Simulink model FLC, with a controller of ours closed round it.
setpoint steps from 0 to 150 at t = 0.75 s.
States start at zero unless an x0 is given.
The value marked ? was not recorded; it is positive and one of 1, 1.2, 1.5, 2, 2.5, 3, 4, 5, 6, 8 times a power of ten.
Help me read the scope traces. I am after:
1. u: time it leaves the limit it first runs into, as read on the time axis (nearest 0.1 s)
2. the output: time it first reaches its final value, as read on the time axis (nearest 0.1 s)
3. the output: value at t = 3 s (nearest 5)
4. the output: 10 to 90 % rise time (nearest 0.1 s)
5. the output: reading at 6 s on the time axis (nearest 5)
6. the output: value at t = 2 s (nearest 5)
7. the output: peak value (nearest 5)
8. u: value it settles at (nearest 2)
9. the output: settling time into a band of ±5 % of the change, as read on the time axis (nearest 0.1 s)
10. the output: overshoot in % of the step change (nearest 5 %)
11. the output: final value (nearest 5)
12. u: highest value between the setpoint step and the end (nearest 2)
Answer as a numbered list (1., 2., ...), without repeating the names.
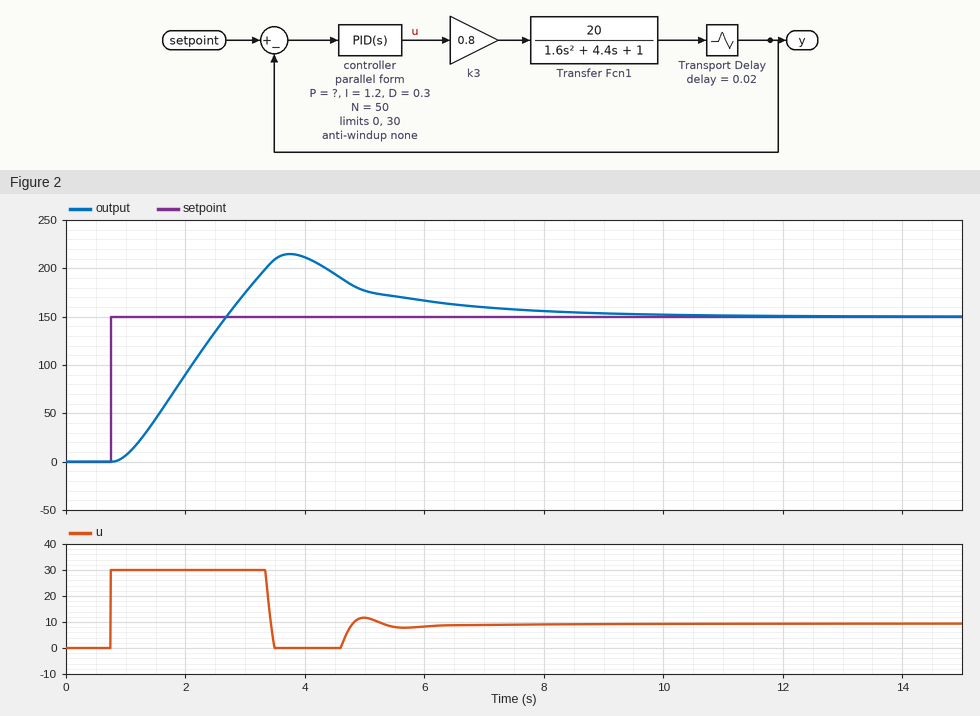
1. 3.3 s
2. 2.7 s
3. 175
4. 1.4 s
5. 165
6. 90
7. 215
8. 10
9. 7.5 s
10. 45 %
11. 150
12. 30
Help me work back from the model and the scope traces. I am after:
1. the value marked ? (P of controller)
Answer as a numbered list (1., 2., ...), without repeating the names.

1. 2.5
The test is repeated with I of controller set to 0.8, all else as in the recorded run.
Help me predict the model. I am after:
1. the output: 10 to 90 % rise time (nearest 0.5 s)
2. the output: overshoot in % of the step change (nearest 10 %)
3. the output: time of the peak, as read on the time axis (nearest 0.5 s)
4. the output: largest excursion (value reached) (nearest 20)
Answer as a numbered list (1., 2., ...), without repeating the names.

1. 1.5 s
2. 30 %
3. 3.5 s
4. 200
